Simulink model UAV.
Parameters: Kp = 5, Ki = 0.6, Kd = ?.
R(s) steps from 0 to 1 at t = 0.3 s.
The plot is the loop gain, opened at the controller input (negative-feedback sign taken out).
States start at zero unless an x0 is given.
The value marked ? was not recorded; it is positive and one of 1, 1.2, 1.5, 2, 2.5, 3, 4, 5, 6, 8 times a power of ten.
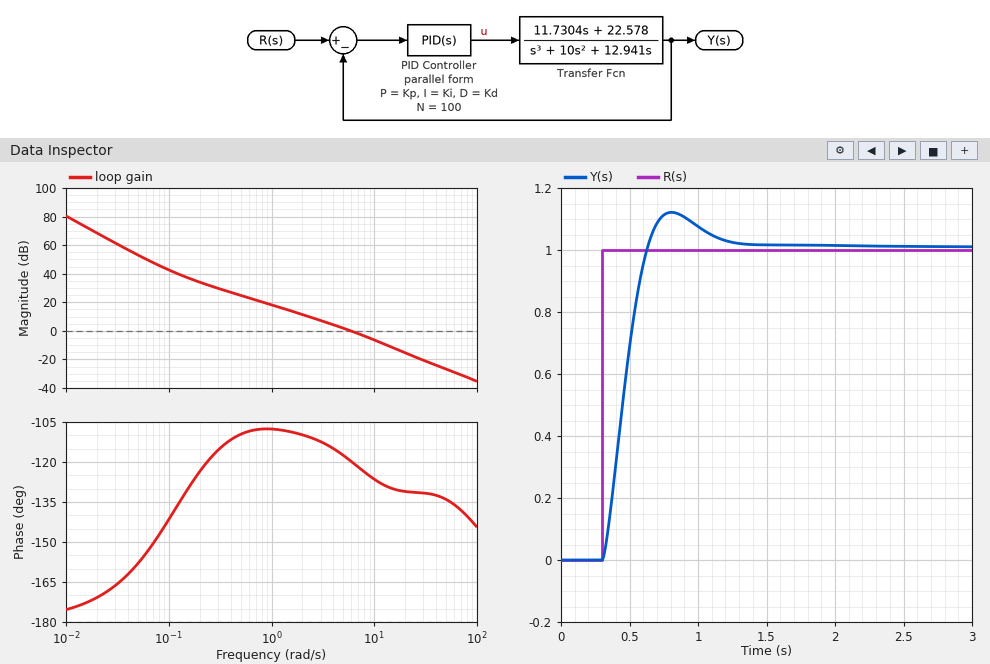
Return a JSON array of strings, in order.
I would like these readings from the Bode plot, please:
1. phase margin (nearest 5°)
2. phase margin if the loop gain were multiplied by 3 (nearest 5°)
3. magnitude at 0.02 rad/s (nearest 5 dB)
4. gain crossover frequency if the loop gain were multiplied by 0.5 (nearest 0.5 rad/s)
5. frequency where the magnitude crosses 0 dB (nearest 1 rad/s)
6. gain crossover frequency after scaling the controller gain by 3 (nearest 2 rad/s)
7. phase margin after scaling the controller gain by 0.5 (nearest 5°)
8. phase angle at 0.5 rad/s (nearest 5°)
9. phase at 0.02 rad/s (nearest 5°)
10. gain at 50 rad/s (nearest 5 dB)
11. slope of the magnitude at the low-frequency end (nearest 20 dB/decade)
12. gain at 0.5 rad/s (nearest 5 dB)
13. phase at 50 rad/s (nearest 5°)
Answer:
["60°", "50°", "70 dB", "3.5 rad/s", "6 rad/s", "12 rad/s", "65°", "-110°", "-170°", "-25 dB", "-40 dB/decade", "25 dB", "-135°"]
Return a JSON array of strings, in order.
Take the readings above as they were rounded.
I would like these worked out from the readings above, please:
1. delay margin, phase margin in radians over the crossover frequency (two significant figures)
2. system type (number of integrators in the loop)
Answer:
["0.17 s", "2"]
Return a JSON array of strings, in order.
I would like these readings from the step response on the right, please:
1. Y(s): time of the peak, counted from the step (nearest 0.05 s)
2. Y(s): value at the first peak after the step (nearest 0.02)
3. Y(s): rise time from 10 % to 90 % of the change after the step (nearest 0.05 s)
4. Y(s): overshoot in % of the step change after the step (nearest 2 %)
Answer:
["0.50 s", "1.12", "0.25 s", "12 %"]
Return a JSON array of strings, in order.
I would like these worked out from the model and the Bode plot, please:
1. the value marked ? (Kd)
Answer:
["0.15"]
